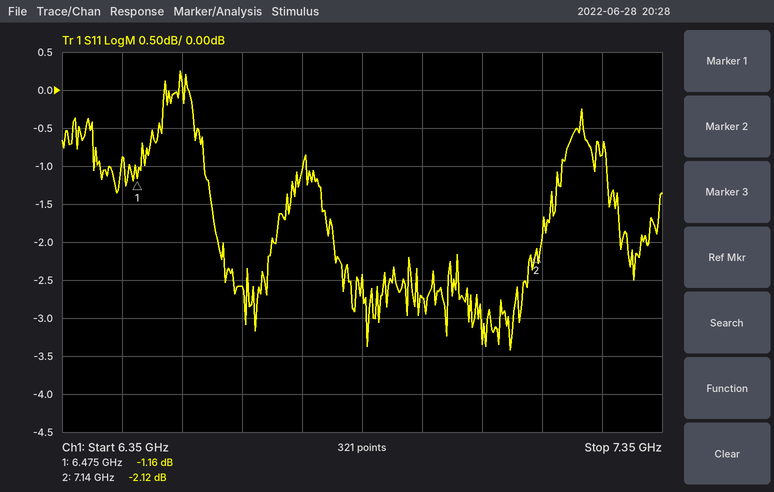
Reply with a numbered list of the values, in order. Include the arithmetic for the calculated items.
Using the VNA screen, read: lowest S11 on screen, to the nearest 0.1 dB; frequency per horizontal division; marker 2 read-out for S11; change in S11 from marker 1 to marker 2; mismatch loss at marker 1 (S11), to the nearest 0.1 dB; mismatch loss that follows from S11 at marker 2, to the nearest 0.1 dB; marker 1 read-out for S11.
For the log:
1. -3.4 dB
2. 100 MHz
3. -2.12 dB
4. -2.12 − (-1.16) = -0.96 dB
5. −10 log10(1 − 10^(-1.16/10)) ≈ 6.3 dB
6. −10 log10(1 − 10^(-2.12/10)) ≈ 4.1 dB
7. -1.16 dB
